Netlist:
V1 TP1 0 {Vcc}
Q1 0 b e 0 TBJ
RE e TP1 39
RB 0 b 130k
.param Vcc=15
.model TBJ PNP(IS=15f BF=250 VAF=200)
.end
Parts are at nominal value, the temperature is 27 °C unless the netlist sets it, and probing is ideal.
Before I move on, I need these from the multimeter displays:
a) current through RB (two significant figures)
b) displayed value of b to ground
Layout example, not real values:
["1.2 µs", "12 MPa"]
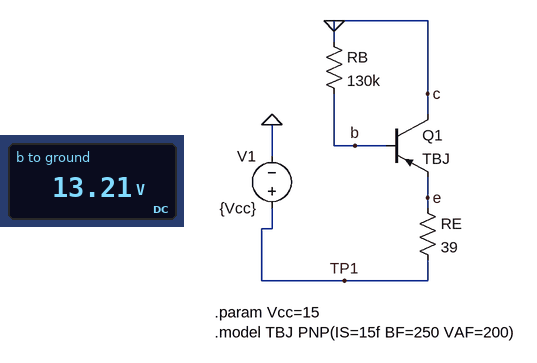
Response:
["100 µA", "13.21 V"]
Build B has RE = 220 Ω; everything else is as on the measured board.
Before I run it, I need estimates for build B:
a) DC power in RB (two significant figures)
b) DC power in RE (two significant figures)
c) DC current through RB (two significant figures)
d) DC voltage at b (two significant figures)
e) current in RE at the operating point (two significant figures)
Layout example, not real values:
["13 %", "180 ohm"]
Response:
["750 µW", "88 mW", "76 µA", "9.9 V", "20 mA"]
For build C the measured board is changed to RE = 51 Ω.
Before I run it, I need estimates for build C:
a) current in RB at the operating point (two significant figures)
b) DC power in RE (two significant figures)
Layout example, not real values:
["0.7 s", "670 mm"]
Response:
["99 µA", "36 mW"]
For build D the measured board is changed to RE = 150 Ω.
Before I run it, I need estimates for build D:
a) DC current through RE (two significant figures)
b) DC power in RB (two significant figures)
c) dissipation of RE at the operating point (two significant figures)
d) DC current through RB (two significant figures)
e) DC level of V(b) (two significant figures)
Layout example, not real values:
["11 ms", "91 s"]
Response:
["22 mA", "920 µW", "74 mW", "84 µA", "11 V"]
